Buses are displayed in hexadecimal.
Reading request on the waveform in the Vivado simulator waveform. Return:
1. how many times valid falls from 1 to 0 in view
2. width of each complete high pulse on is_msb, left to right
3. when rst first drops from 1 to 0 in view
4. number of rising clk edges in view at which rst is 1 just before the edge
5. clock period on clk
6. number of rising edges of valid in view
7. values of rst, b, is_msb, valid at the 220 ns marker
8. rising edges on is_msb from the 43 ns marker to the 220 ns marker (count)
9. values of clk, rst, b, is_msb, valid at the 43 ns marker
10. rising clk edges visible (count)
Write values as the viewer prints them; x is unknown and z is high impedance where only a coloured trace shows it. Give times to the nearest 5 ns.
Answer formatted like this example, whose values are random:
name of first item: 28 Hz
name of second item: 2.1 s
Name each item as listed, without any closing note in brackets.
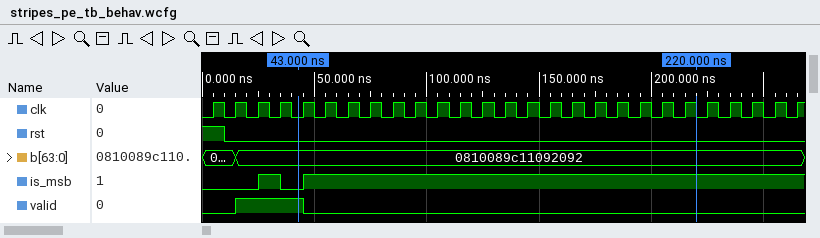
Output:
how many times valid falls from 1 to 0 in view: 1
width of each complete high pulse on is_msb, left to right: 10 ns
when rst first drops from 1 to 0 in view: 10 ns
number of rising clk edges in view at which rst is 1 just before the edge: 1
clock period on clk: 10 ns
number of rising edges of valid in view: 1
values of rst, b, is_msb, valid at the 220 ns marker: rst=0, b=0810089c11092092, is_msb=1, valid=0
rising edges on is_msb from the 43 ns marker to the 220 ns marker: 1
values of clk, rst, b, is_msb, valid at the 43 ns marker: clk=0, rst=0, b=0810089c11092092, is_msb=0, valid=1
rising clk edges visible: 27
